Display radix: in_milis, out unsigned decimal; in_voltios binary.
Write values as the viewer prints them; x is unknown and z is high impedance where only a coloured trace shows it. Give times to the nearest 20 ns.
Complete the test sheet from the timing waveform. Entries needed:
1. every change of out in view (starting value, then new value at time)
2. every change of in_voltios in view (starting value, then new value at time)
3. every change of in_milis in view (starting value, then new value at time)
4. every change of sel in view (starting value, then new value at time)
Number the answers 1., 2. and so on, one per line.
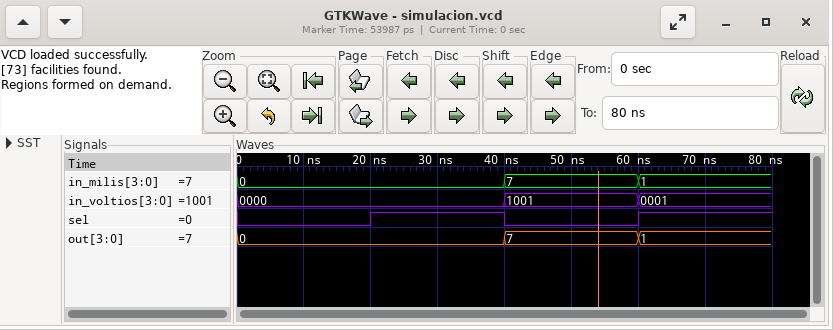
1. 0, 7 at 40 ns, 1 at 60 ns
2. 0000, 1001 at 40 ns, 0001 at 60 ns
3. 0, 7 at 40 ns, 1 at 60 ns
4. 0, 1 at 20 ns, 0 at 40 ns, 1 at 60 ns
